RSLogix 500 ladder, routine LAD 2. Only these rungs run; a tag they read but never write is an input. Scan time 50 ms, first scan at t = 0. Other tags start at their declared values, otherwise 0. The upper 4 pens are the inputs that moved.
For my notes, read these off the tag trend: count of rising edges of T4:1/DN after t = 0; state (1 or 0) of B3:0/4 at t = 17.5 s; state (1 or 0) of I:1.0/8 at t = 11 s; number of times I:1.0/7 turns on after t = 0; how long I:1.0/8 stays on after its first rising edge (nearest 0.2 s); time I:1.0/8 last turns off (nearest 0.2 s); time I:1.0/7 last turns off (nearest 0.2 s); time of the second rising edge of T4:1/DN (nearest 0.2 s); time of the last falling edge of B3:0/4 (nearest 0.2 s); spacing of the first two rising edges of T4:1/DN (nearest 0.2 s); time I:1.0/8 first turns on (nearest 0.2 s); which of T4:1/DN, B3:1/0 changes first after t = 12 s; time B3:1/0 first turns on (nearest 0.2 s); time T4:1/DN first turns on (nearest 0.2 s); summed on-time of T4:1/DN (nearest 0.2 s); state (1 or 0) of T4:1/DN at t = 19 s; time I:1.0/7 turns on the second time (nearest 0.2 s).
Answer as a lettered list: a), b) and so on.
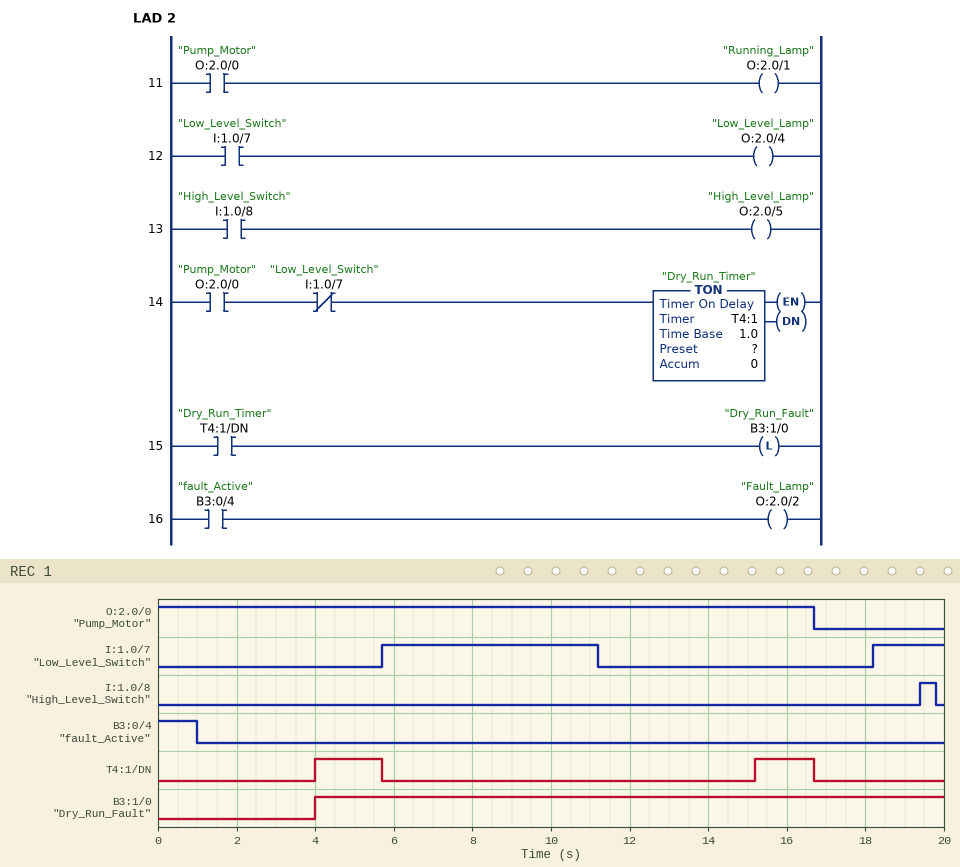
a) 2
b) 0
c) 0
d) 2
e) 0.4 s
f) 19.8 s
g) 11.2 s
h) 15.2 s
i) 1.0 s
j) 11.2 s
k) 19.4 s
l) T4:1/DN
m) 4.0 s
n) 4.0 s
o) 3.2 s
p) 0
q) 18.2 s
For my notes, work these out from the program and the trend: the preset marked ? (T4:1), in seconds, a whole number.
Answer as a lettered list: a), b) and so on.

a) 4 s
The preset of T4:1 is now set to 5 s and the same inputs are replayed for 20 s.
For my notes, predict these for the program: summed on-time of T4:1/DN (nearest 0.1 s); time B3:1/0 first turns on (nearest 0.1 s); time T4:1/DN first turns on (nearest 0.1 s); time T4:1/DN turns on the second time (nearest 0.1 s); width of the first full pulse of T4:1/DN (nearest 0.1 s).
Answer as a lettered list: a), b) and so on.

a) 1.2 s
b) 5.0 s
c) 5.0 s
d) 16.2 s
e) 0.7 s
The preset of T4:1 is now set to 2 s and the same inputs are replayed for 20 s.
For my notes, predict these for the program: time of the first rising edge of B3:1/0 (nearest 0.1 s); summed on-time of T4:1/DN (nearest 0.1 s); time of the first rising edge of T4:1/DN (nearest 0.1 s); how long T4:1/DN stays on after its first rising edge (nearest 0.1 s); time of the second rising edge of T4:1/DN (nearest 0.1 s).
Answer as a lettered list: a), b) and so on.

a) 2.0 s
b) 7.2 s
c) 2.0 s
d) 3.7 s
e) 13.2 s
